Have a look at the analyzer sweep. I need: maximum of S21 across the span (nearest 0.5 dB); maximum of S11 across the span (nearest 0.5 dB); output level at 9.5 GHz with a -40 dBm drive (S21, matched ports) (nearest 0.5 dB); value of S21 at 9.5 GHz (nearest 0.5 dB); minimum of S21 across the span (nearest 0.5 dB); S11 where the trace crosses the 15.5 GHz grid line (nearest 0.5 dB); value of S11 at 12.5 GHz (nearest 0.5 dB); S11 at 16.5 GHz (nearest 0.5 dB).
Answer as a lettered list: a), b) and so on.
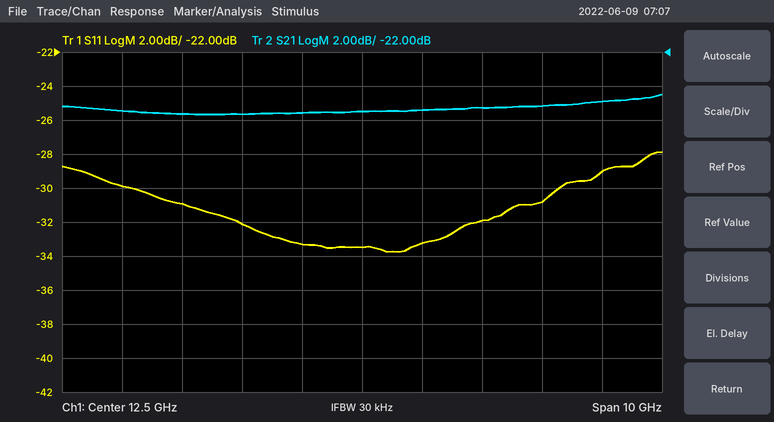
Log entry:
a) -24.5 dB
b) -28.0 dB
c) -65.5 dBm
d) -25.5 dB
e) -25.5 dB
f) -31.0 dB
g) -33.5 dB
h) -29.0 dB
